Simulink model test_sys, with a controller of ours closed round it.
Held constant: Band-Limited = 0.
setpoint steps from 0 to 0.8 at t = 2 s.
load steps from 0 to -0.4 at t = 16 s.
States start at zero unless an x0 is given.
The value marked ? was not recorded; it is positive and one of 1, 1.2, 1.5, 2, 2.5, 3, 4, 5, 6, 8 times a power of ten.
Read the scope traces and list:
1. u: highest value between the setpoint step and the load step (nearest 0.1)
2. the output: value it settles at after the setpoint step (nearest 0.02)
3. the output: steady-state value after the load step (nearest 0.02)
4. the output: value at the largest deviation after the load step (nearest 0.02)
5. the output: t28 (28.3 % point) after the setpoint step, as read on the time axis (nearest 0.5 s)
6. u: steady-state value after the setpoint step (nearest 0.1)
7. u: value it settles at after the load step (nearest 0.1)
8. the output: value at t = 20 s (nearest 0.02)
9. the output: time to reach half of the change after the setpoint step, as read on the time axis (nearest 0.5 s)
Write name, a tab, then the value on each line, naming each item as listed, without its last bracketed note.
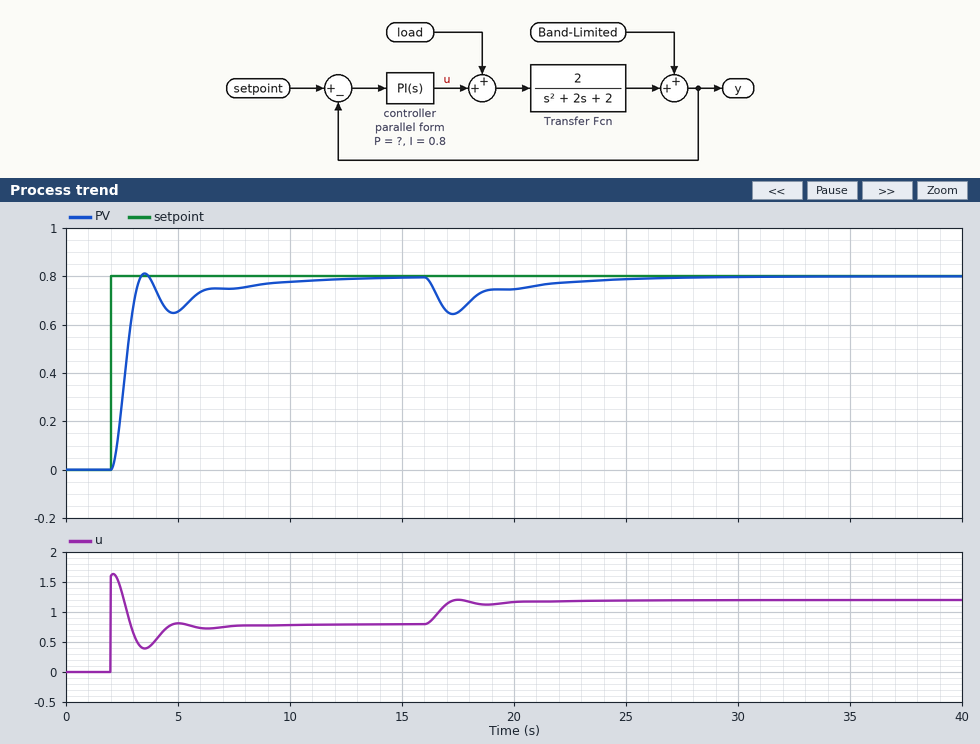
u: highest value between the setpoint step and the load step	1.6
the output: value it settles at after the setpoint step	0.80
the output: steady-state value after the load step	0.80
the output: value at the largest deviation after the load step	0.64
the output: t28 (28.3 % point) after the setpoint step, as read on the time axis	2.5 s
u: steady-state value after the setpoint step	0.8
u: value it settles at after the load step	1.2
the output: value at t = 20 s	0.74
the output: time to reach half of the change after the setpoint step, as read on the time axis	2.5 s
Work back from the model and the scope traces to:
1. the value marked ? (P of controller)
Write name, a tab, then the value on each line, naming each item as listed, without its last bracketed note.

the value marked ?	2
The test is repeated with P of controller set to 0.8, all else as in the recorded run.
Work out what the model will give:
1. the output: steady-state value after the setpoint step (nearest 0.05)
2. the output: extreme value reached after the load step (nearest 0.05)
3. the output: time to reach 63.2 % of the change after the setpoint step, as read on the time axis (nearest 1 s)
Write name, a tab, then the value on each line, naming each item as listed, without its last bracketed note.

the output: steady-state value after the setpoint step	0.80
the output: extreme value reached after the load step	0.60
the output: time to reach 63.2 % of the change after the setpoint step, as read on the time axis	3 s
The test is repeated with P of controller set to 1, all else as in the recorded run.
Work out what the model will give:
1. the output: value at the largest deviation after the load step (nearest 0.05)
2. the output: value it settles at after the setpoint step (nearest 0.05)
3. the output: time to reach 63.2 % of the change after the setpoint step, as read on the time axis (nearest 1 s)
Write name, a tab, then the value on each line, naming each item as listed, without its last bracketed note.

the output: value at the largest deviation after the load step	0.60
the output: value it settles at after the setpoint step	0.80
the output: time to reach 63.2 % of the change after the setpoint step, as read on the time axis	3 s
